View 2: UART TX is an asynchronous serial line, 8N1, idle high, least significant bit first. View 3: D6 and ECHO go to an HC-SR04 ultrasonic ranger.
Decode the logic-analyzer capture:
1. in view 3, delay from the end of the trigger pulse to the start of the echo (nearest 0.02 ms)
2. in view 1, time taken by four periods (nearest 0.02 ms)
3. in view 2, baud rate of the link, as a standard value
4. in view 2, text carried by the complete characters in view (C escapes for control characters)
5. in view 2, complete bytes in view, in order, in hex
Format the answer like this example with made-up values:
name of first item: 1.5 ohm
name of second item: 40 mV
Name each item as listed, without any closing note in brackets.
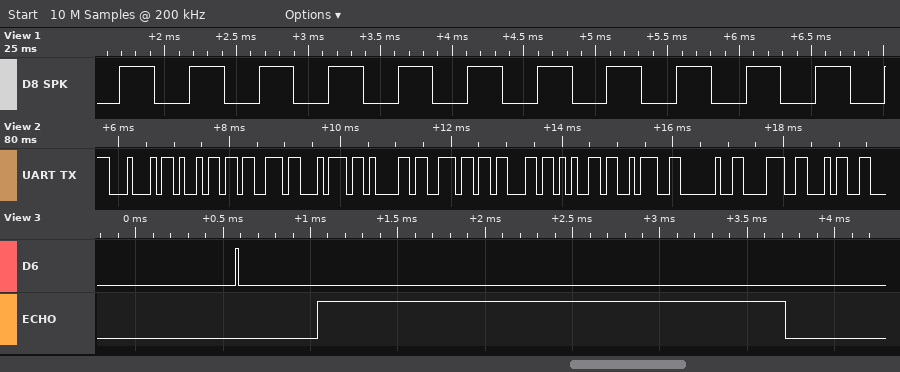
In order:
in view 3, delay from the end of the trigger pulse to the start of the echo: 0.46 ms
in view 1, time taken by four periods: 1.94 ms
in view 2, baud rate of the link, as a standard value: 9600 baud
in view 2, text carried by the complete characters in view: "Distance: 84"
in view 2, complete bytes in view, in order, in hex: 44 69 73 74 61 6E 63 65 3A 20 38 34
